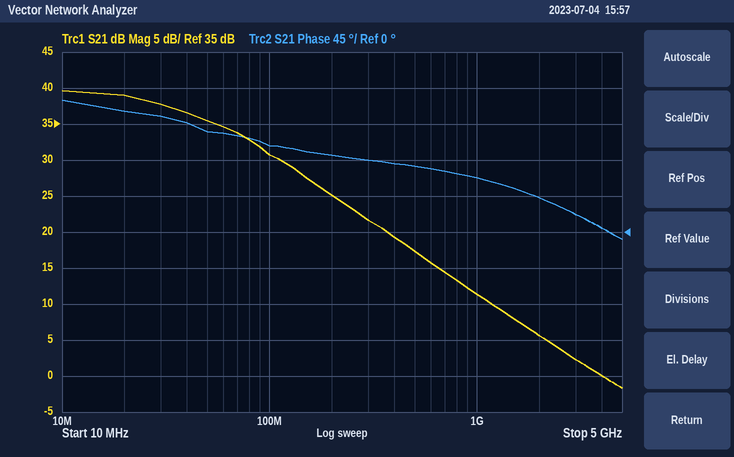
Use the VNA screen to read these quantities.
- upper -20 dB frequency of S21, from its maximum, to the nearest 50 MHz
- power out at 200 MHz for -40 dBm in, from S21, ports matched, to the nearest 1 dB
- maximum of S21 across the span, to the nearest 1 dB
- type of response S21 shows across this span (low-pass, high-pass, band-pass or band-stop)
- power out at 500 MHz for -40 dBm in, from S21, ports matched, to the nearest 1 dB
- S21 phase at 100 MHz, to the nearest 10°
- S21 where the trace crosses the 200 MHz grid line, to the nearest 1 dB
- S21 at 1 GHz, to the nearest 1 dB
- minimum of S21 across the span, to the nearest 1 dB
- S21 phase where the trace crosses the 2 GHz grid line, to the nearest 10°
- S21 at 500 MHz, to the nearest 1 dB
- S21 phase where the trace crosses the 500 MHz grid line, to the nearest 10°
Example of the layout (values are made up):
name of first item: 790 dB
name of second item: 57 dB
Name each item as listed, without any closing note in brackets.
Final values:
upper -20 dB frequency of S21, from its maximum, to the nearest 50 MHz: 400 MHz
power out at 200 MHz for -40 dBm in, from S21, ports matched, to the nearest 1 dB: -15 dBm
maximum of S21 across the span, to the nearest 1 dB: 40 dB
type of response S21 shows across this span: low-pass
power out at 500 MHz for -40 dBm in, from S21, ports matched, to the nearest 1 dB: -23 dBm
S21 phase at 100 MHz, to the nearest 10°: 110°
S21 where the trace crosses the 200 MHz grid line, to the nearest 1 dB: 25 dB
S21 at 1 GHz, to the nearest 1 dB: 11 dB
minimum of S21 across the span, to the nearest 1 dB: -2 dB
S21 phase where the trace crosses the 2 GHz grid line, to the nearest 10°: 40°
S21 at 500 MHz, to the nearest 1 dB: 17 dB
S21 phase where the trace crosses the 500 MHz grid line, to the nearest 10°: 80°
